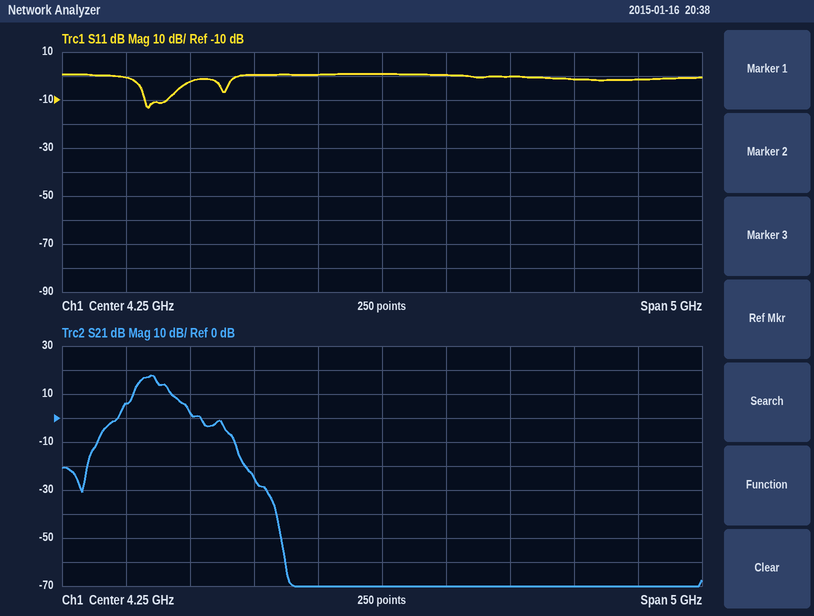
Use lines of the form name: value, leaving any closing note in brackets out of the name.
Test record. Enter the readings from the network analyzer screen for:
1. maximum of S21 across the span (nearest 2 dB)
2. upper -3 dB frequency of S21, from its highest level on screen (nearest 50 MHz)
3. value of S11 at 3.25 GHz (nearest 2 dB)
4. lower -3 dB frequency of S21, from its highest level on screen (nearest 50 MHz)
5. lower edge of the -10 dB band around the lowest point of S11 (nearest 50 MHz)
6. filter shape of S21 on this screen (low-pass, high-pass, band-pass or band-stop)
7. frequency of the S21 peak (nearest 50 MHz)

maximum of S21 across the span: 18 dB
upper -3 dB frequency of S21, from its highest level on screen: 2.50 GHz
value of S11 at 3.25 GHz: 0 dB
lower -3 dB frequency of S21, from its highest level on screen: 2.35 GHz
lower edge of the -10 dB band around the lowest point of S11: 2.40 GHz
filter shape of S21 on this screen: band-pass
frequency of the S21 peak: 2.45 GHz
